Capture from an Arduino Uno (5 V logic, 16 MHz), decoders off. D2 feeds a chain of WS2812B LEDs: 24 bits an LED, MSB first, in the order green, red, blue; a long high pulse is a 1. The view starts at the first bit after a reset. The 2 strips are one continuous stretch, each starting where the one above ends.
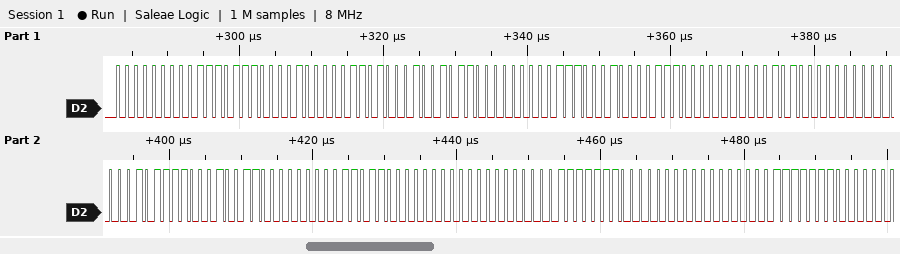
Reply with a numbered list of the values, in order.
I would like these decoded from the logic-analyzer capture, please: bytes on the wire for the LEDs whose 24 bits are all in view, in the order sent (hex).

1. 00 77 08 34 4B 00 71 0E 00 50 00 2F 13 00 6C 00 00 7F 00 00 7F
